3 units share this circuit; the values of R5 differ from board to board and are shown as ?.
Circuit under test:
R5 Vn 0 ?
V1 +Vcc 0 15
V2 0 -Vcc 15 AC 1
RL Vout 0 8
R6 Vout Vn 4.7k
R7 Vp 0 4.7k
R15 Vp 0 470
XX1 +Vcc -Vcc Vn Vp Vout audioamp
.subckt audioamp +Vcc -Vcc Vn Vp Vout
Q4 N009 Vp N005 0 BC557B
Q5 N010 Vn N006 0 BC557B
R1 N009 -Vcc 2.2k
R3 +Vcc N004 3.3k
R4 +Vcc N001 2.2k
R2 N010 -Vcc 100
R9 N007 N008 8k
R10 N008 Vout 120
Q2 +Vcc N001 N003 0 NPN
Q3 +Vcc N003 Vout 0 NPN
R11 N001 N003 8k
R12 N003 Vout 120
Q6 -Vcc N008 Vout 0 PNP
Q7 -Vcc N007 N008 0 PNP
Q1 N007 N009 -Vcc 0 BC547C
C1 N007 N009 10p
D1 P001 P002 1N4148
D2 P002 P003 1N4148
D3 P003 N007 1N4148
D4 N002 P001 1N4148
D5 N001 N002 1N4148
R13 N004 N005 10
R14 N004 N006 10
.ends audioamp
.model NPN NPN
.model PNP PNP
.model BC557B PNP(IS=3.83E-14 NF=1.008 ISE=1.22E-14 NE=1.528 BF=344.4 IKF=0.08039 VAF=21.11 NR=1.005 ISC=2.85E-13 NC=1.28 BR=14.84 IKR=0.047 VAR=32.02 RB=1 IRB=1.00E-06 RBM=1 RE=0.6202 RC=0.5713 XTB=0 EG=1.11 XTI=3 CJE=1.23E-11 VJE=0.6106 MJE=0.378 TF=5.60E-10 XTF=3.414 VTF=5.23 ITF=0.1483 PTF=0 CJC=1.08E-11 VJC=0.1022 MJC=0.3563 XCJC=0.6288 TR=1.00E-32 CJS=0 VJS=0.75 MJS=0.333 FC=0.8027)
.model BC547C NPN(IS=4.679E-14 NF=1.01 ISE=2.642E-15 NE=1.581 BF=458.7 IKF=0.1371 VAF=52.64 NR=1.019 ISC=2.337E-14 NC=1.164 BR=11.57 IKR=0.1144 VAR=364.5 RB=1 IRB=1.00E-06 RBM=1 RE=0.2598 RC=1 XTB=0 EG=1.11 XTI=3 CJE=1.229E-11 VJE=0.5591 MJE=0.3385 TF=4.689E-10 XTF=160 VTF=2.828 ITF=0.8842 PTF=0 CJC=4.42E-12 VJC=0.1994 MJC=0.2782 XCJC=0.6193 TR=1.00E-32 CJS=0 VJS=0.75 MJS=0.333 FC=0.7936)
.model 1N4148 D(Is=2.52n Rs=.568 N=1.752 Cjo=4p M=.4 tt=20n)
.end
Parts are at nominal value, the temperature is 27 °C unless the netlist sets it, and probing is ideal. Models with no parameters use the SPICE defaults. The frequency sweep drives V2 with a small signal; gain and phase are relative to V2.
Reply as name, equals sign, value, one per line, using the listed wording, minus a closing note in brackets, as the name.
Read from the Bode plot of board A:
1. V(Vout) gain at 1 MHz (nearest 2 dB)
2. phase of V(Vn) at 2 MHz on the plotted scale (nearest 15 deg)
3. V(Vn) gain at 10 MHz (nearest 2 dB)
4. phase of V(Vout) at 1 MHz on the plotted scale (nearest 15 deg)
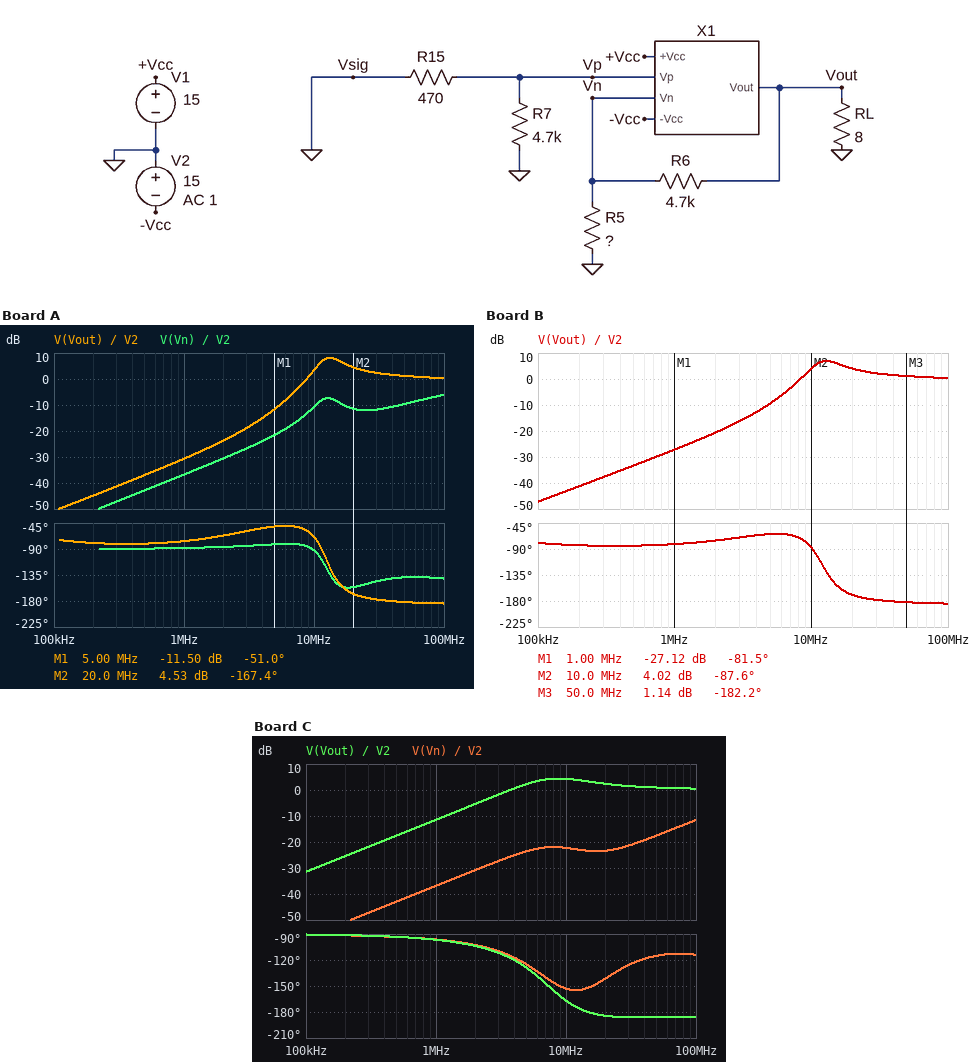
V(Vout) gain at 1 MHz = -30 dB
phase of V(Vn) at 2 MHz on the plotted scale = -90 deg
V(Vn) gain at 10 MHz = -10 dB
phase of V(Vout) at 1 MHz on the plotted scale = -75 deg
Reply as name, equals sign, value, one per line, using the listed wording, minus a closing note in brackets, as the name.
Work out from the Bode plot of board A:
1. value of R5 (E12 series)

value of R5 = 1 kΩ
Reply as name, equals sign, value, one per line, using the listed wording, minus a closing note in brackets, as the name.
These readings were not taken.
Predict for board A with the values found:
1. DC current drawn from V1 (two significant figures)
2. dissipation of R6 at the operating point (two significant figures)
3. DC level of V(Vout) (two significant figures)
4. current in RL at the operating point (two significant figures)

DC current drawn from V1 = 22 mA
dissipation of R6 at the operating point = 61 µW
DC level of V(Vout) = -640 mV
current in RL at the operating point = 80 mA
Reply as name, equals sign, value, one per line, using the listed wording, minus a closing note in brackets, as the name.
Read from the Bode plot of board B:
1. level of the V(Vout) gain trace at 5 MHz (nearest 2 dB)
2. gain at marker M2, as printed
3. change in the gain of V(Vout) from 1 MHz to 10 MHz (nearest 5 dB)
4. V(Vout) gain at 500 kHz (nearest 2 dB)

level of the V(Vout) gain trace at 5 MHz = -10 dB
gain at marker M2, as printed = 4.02 dB
change in the gain of V(Vout) from 1 MHz to 10 MHz = 30 dB
V(Vout) gain at 500 kHz = -34 dB
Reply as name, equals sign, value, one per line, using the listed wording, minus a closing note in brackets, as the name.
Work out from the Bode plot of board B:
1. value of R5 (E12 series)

value of R5 = 820 Ω
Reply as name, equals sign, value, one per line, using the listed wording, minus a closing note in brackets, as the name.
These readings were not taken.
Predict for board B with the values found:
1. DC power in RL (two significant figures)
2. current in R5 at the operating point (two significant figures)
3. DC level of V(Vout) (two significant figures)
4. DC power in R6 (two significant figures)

DC power in RL = 71 mW
current in R5 at the operating point = 130 µA
DC level of V(Vout) = -750 mV
DC power in R6 = 89 µW
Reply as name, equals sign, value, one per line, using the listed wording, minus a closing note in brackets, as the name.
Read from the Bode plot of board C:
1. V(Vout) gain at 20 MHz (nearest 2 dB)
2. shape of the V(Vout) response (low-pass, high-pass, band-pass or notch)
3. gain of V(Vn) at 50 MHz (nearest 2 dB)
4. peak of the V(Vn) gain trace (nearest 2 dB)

V(Vout) gain at 20 MHz = 2 dB
shape of the V(Vout) response = high-pass
gain of V(Vn) at 50 MHz = -18 dB
peak of the V(Vn) gain trace = -12 dB
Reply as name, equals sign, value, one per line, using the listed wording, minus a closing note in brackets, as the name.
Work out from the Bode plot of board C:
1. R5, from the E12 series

R5, from the E12 series = 220 Ω
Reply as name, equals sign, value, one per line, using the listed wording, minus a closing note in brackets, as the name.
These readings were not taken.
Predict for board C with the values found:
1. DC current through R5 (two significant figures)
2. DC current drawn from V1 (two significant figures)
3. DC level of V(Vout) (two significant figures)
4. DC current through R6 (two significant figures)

DC current through R5 = 480 µA
DC current drawn from V1 = 21 mA
DC level of V(Vout) = -2.4 V
DC current through R6 = 490 µA
